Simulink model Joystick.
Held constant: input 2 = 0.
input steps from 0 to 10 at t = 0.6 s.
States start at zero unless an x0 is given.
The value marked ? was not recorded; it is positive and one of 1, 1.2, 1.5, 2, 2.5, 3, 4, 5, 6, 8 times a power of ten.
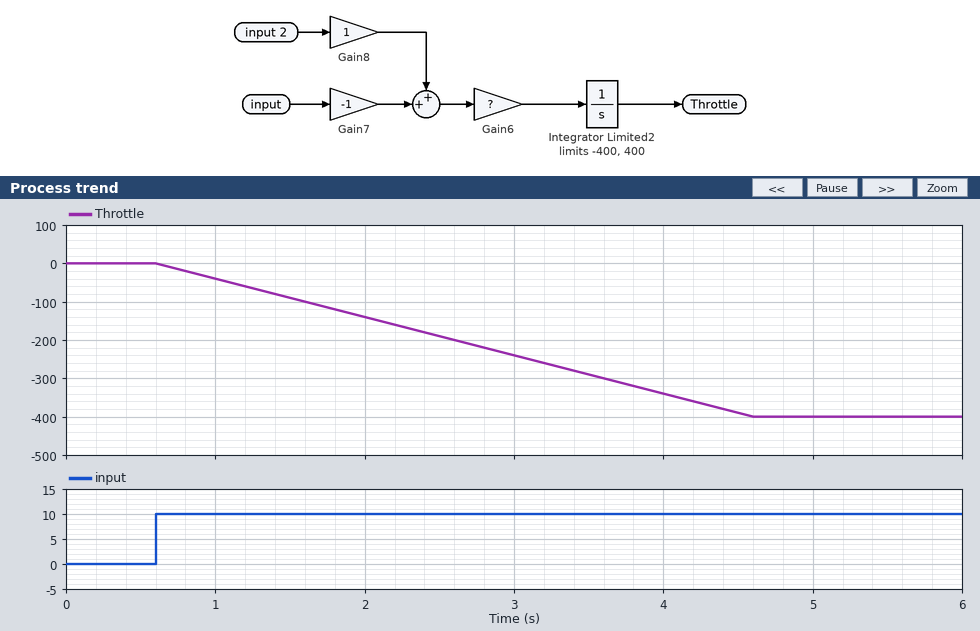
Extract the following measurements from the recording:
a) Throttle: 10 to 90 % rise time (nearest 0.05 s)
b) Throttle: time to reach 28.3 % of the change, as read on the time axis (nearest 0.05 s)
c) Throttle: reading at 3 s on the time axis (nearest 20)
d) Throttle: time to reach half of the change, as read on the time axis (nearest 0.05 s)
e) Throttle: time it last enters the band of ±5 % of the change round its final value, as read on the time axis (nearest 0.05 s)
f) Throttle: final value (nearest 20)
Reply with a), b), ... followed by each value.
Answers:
a) 3.20 s
b) 1.75 s
c) -240
d) 2.60 s
e) 4.40 s
f) -400
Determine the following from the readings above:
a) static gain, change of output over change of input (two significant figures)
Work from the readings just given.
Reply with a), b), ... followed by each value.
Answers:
a) -40
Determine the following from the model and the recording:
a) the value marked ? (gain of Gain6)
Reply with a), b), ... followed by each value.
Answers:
a) 10
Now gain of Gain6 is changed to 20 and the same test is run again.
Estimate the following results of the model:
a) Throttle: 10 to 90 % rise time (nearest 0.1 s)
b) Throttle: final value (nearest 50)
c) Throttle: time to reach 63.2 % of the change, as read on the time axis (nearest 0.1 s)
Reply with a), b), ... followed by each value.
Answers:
a) 1.6 s
b) -400
c) 1.9 s
